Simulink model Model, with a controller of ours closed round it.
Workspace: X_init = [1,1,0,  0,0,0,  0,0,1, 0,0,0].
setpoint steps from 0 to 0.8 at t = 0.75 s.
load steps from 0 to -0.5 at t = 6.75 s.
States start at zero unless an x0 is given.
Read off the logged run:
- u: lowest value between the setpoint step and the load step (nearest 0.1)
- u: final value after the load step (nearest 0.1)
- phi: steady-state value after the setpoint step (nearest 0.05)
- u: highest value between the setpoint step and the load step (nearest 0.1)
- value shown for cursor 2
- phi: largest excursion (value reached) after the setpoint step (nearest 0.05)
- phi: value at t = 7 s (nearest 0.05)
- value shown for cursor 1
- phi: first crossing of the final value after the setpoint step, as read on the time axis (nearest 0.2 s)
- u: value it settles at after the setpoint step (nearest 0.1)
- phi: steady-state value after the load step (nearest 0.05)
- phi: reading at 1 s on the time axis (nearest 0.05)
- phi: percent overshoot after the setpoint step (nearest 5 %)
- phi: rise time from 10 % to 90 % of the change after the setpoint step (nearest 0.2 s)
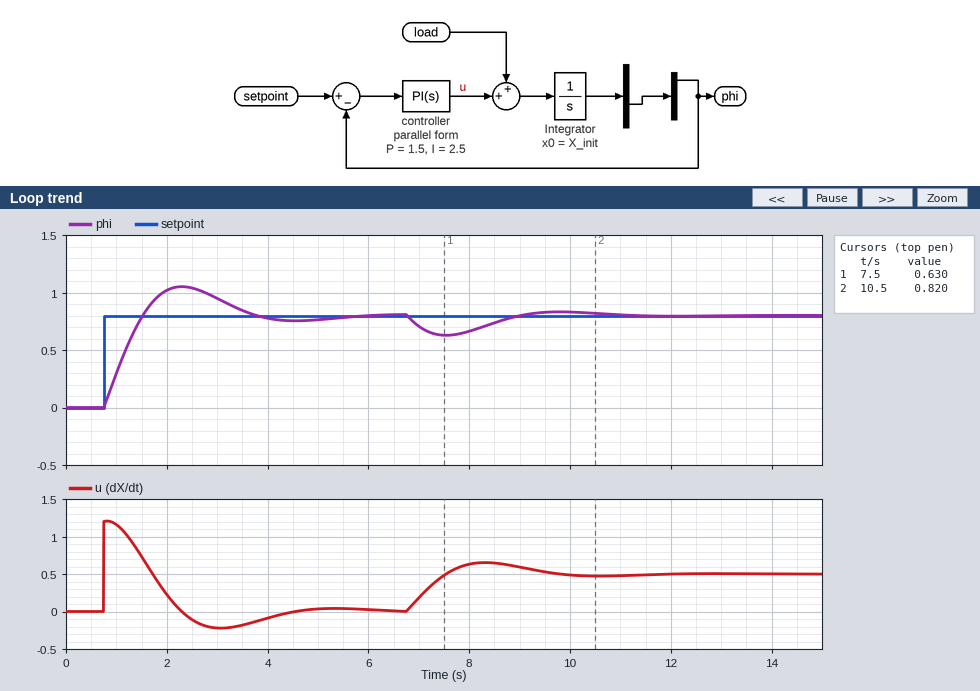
-0.2
0.5
0.80
1.2
0.820
1.05
0.70
0.630
1.6 s
0.0
0.80
0.30
30 %
0.6 s
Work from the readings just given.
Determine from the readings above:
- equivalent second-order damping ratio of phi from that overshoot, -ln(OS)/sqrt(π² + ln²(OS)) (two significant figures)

0.36
